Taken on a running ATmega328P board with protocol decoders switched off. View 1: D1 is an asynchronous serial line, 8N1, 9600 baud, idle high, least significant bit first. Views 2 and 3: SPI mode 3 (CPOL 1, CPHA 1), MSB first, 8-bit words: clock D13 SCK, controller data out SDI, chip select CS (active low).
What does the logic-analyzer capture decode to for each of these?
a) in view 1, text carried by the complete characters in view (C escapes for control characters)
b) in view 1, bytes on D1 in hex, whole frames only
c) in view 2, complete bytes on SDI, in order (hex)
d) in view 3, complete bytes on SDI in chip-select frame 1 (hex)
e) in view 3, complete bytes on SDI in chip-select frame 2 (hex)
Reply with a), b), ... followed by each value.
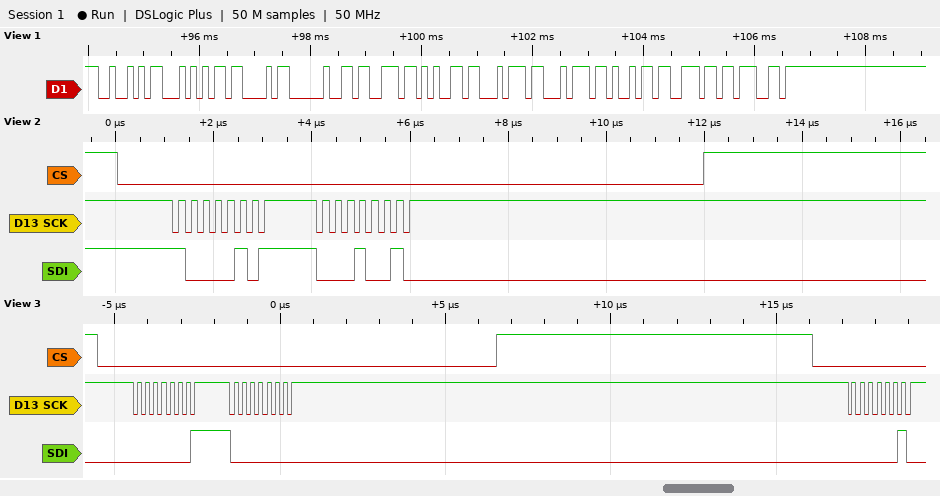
a) "RTC setting"
b) 52 54 43 20 73 65 74 74 69 6E 67
c) 85 12
d) 01 00
e) 02
